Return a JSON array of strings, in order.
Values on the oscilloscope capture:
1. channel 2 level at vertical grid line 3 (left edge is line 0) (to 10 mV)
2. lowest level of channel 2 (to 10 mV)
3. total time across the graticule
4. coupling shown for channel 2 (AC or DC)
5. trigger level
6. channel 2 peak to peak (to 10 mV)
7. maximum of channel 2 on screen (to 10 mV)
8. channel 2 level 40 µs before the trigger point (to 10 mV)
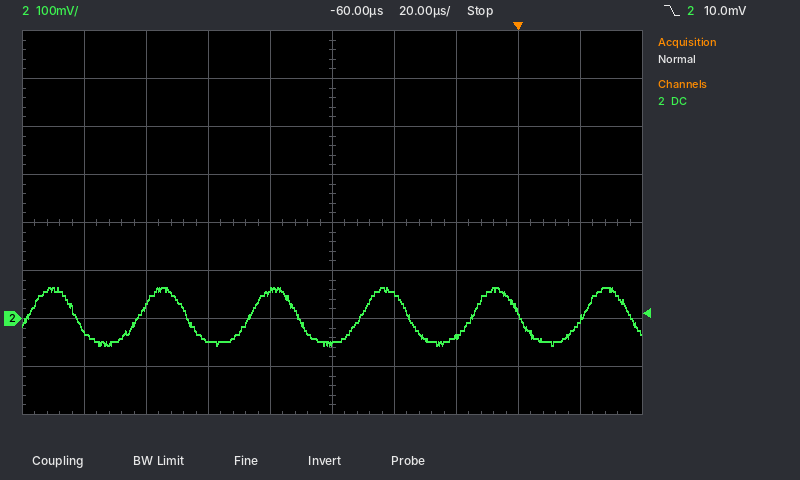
["-50 mV", "-60 mV", "200 µs", "DC", "10.0 mV", "120 mV", "60 mV", "50 mV"]
